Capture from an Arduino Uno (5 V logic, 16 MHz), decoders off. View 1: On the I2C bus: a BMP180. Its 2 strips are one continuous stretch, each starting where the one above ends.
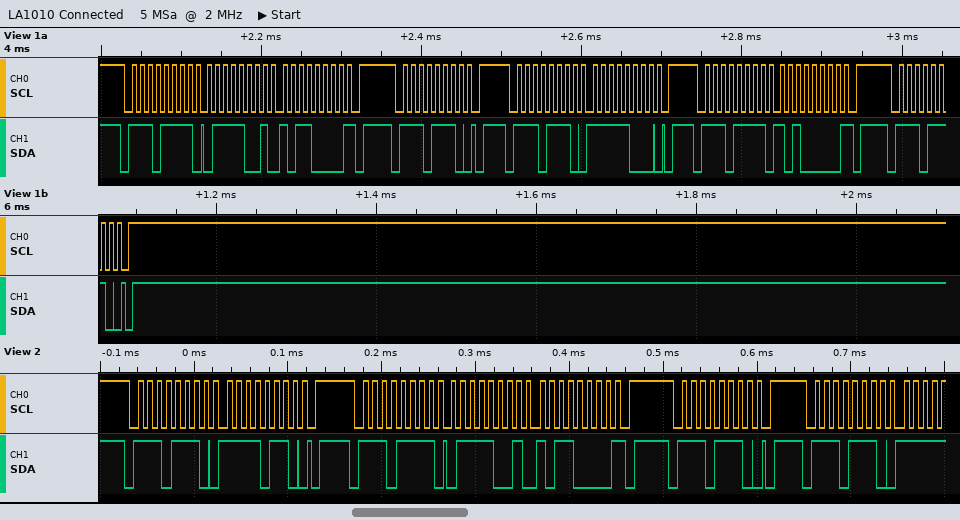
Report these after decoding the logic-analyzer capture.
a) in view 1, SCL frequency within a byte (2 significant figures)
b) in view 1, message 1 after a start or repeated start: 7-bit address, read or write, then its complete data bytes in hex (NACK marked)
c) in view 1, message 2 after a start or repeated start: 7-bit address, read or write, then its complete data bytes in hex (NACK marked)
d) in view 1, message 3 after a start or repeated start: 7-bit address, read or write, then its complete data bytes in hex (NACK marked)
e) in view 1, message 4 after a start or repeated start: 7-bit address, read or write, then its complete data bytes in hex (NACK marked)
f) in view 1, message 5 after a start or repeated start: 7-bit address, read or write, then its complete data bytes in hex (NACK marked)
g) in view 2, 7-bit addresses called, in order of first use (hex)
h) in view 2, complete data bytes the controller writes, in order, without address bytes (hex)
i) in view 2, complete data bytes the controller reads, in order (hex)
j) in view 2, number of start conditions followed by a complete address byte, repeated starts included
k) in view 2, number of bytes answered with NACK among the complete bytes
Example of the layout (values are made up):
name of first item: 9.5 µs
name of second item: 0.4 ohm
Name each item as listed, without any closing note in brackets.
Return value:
in view 1, SCL frequency within a byte: 100 kHz
in view 1, message 1 after a start or repeated start: 7-bit address, read or write, then its complete data bytes in hex: 0x77 read: 79 B0 NACK
in view 1, message 2 after a start or repeated start: 7-bit address, read or write, then its complete data bytes in hex: 0x77 write
in view 1, message 3 after a start or repeated start: 7-bit address, read or write, then its complete data bytes in hex: 0x77 write: F8
in view 1, message 4 after a start or repeated start: 7-bit address, read or write, then its complete data bytes in hex: 0x77 read: A0 NACK
in view 1, message 5 after a start or repeated start: 7-bit address, read or write, then its complete data bytes in hex: 0x77 write
in view 2, 7-bit addresses called, in order of first use: 0x77
in view 2, complete data bytes the controller writes, in order, without address bytes: F6
in view 2, complete data bytes the controller reads, in order: 79 B0
in view 2, number of start conditions followed by a complete address byte, repeated starts included: 4
in view 2, number of bytes answered with NACK among the complete bytes: 1
